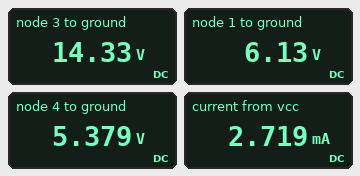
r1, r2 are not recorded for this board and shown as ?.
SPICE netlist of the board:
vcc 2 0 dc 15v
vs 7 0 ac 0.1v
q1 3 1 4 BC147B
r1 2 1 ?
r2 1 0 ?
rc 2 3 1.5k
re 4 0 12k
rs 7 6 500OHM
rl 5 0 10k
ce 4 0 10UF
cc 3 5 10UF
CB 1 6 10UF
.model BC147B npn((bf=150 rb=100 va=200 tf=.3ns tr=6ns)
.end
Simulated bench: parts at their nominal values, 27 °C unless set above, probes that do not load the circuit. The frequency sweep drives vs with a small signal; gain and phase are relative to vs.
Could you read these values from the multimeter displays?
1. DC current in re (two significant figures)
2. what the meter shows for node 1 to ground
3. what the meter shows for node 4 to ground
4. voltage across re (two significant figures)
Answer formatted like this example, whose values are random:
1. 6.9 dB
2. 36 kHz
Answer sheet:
1. 450 µA
2. 6.13 V
3. 5.379 V
4. 5.4 V
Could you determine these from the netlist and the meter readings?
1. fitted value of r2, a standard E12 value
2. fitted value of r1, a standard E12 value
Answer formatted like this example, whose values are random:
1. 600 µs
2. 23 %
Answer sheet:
1. 2.7 kΩ
2. 3.9 kΩ
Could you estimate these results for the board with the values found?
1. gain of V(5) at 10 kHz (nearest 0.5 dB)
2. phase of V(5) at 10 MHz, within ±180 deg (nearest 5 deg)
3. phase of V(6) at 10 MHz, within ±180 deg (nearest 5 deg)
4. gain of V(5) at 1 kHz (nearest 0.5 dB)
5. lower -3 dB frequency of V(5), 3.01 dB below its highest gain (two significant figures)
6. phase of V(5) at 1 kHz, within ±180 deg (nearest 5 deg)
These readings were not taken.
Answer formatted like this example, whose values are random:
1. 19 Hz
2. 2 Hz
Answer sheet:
1. 24.0 dB
2. 170 deg
3. -5 deg
4. 24.0 dB
5. 260 Hz
6. -165 deg
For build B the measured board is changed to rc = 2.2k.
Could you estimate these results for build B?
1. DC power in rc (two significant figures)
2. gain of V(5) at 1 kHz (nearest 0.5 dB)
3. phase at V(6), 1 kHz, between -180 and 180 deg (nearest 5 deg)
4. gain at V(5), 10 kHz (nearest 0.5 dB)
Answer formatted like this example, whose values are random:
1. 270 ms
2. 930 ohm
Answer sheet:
1. 440 µW
2. 26.5 dB
3. 0 deg
4. 27.0 dB
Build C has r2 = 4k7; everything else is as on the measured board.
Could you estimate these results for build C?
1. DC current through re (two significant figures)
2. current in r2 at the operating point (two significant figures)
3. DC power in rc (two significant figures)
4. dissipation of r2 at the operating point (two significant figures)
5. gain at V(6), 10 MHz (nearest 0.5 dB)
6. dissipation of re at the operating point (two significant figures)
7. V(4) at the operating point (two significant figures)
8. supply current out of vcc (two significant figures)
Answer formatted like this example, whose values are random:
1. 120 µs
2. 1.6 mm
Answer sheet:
1. 620 µA
2. 1.7 mA
3. 570 µW
4. 14 mW
5. -2.5 dB
6. 4.6 mW
7. 7.4 V
8. 2.4 mA
